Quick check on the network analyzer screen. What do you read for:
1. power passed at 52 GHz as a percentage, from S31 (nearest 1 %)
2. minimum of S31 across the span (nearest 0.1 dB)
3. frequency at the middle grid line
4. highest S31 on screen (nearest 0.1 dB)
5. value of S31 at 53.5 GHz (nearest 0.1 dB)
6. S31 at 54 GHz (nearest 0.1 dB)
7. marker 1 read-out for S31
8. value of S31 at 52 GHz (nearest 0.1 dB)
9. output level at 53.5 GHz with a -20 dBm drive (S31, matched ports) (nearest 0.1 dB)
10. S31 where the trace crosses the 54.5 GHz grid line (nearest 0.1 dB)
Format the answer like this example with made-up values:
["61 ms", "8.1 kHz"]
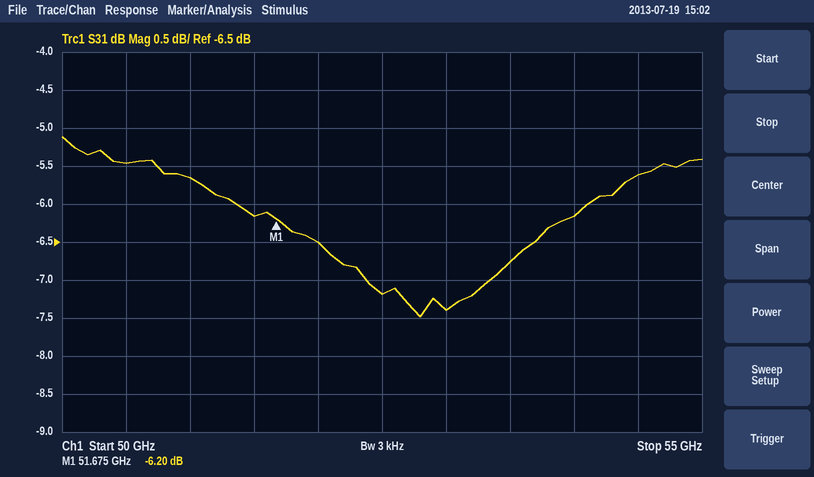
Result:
["22 %", "-7.5 dB", "52.5 GHz", "-5.1 dB", "-6.8 dB", "-6.2 dB", "-6.20 dB", "-6.5 dB", "-26.8 dBm", "-5.6 dB"]
